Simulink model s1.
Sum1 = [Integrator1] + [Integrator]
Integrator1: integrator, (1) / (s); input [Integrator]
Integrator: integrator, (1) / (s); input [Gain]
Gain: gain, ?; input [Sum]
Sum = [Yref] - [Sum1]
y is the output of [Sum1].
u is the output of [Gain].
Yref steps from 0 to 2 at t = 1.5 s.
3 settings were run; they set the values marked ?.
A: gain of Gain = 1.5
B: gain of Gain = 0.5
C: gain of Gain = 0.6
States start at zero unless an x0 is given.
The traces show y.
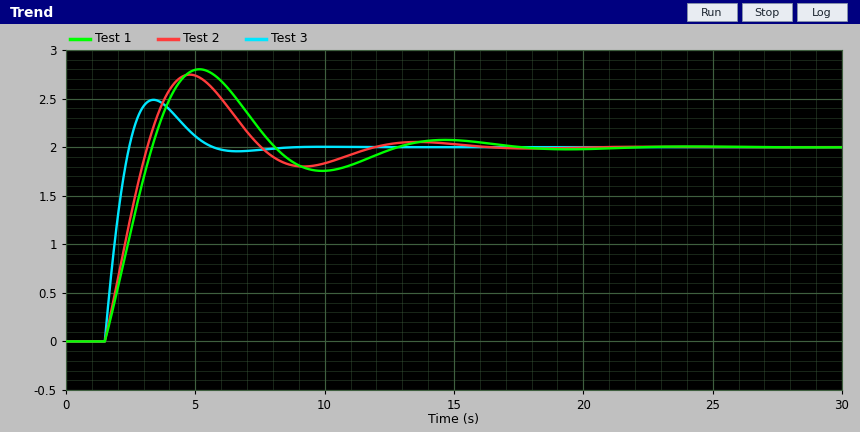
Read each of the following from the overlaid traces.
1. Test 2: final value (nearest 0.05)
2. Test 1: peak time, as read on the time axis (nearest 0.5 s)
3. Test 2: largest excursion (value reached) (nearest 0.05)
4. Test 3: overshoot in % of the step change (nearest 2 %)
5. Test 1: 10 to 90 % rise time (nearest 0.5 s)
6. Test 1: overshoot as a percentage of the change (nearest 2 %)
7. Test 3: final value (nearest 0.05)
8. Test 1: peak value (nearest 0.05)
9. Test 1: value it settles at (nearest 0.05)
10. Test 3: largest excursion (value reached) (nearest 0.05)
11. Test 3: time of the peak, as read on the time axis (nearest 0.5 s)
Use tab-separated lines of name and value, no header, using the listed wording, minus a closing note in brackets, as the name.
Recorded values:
Test 2: final value	2.00
Test 1: peak time, as read on the time axis	5.0 s
Test 2: largest excursion (value reached)	2.75
Test 3: overshoot in % of the step change	24 %
Test 1: 10 to 90 % rise time	1.5 s
Test 1: overshoot as a percentage of the change	40 %
Test 3: final value	2.00
Test 1: peak value	2.80
Test 1: value it settles at	2.00
Test 3: largest excursion (value reached)	2.50
Test 3: time of the peak, as read on the time axis	3.5 s
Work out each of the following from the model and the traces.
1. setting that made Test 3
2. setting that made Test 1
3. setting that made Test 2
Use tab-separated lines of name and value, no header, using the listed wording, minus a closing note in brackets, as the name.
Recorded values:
setting that made Test 3	A
setting that made Test 1	B
setting that made Test 2	C
